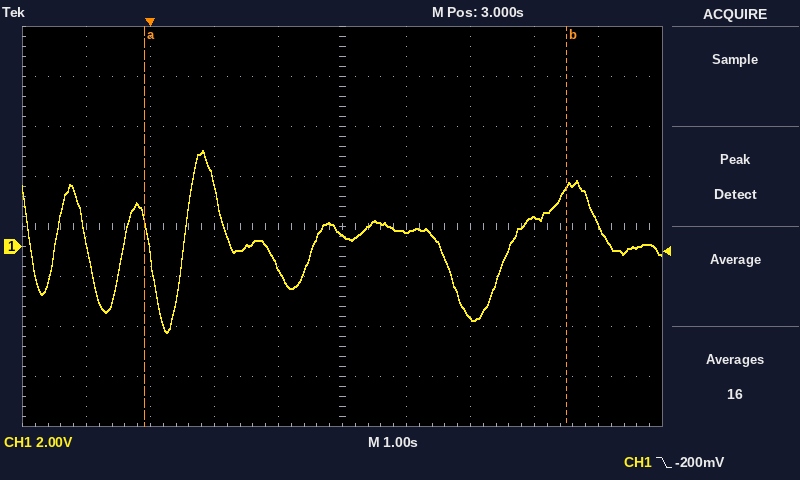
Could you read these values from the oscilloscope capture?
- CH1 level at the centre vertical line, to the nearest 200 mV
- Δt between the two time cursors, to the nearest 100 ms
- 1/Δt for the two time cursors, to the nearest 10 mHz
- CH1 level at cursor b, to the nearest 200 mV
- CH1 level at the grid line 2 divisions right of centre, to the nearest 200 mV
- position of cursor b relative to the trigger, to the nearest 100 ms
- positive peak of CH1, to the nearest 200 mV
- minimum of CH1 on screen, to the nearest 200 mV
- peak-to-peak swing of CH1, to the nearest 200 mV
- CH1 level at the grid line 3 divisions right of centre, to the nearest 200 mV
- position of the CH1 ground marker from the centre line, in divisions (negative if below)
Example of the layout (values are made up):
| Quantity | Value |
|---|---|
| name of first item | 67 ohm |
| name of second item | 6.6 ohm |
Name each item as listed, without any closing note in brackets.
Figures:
| Quantity | Value |
|---|---|
| CH1 level at the centre vertical line, to the nearest 200 mV | 400 mV |
| Δt between the two time cursors, to the nearest 100 ms | 6.6 s |
| 1/Δt for the two time cursors, to the nearest 10 mHz | 150 mHz |
| CH1 level at cursor b, to the nearest 200 mV | 2.4 V |
| CH1 level at the grid line 2 divisions right of centre, to the nearest 200 mV | -2.8 V |
| position of cursor b relative to the trigger, to the nearest 100 ms | +6.5 s |
| positive peak of CH1, to the nearest 200 mV | 3.8 V |
| minimum of CH1 on screen, to the nearest 200 mV | -3.4 V |
| peak-to-peak swing of CH1, to the nearest 200 mV | 7.2 V |
| CH1 level at the grid line 3 divisions right of centre, to the nearest 200 mV | 1.2 V |
| position of the CH1 ground marker from the centre line, in divisions | -0.4 div |
